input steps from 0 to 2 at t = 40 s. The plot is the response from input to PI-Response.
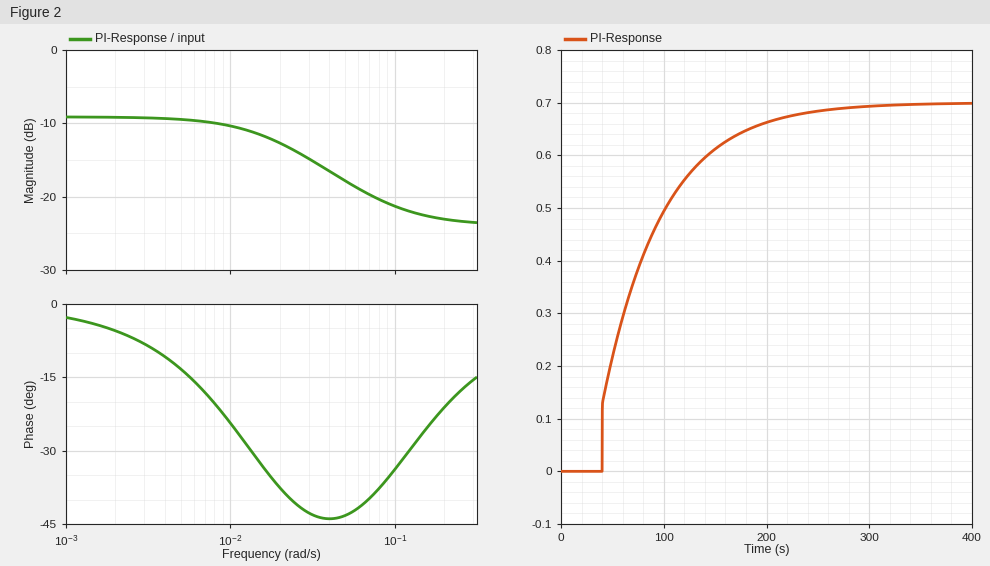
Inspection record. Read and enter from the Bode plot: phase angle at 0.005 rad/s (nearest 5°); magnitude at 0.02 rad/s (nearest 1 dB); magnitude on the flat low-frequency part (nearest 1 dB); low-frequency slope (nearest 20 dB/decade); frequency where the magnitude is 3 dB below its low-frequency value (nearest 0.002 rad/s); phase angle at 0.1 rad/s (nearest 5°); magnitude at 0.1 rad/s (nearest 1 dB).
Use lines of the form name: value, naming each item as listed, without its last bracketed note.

phase angle at 0.005 rad/s: -15°
magnitude at 0.02 rad/s: -13 dB
magnitude on the flat low-frequency part: -9 dB
low-frequency slope: 0 dB/decade
frequency where the magnitude is 3 dB below its low-frequency value: 0.018 rad/s
phase angle at 0.1 rad/s: -35°
magnitude at 0.1 rad/s: -21 dB
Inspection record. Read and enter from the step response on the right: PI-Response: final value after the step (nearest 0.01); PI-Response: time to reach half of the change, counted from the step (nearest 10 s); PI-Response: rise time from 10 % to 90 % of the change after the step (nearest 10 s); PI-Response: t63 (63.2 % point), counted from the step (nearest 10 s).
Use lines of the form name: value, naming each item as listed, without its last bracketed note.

PI-Response: final value after the step: 0.70
PI-Response: time to reach half of the change, counted from the step: 30 s
PI-Response: rise time from 10 % to 90 % of the change after the step: 120 s
PI-Response: t63 (63.2 % point), counted from the step: 50 s
